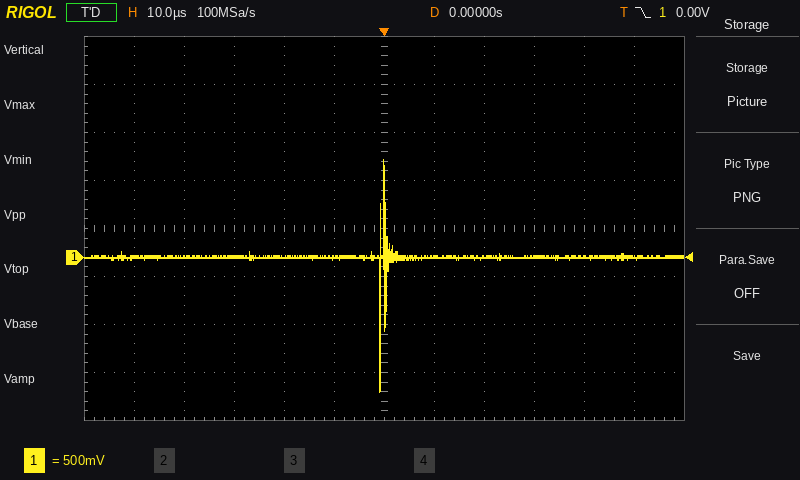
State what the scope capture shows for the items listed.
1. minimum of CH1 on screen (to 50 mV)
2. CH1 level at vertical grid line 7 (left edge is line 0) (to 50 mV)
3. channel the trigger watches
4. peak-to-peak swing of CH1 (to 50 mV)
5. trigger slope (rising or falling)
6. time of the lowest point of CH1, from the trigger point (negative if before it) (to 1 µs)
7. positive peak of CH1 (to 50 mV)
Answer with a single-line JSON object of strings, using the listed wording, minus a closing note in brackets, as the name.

{"minimum of CH1 on screen": "-1.40 V", "CH1 level at vertical grid line 7 (left edge is line 0)": "0 mV", "channel the trigger watches": "CH1", "peak-to-peak swing of CH1": "2.40 V", "trigger slope": "falling", "time of the lowest point of CH1, from the trigger point (negative if before it)": "-1 µs", "positive peak of CH1": "1.00 V"}
